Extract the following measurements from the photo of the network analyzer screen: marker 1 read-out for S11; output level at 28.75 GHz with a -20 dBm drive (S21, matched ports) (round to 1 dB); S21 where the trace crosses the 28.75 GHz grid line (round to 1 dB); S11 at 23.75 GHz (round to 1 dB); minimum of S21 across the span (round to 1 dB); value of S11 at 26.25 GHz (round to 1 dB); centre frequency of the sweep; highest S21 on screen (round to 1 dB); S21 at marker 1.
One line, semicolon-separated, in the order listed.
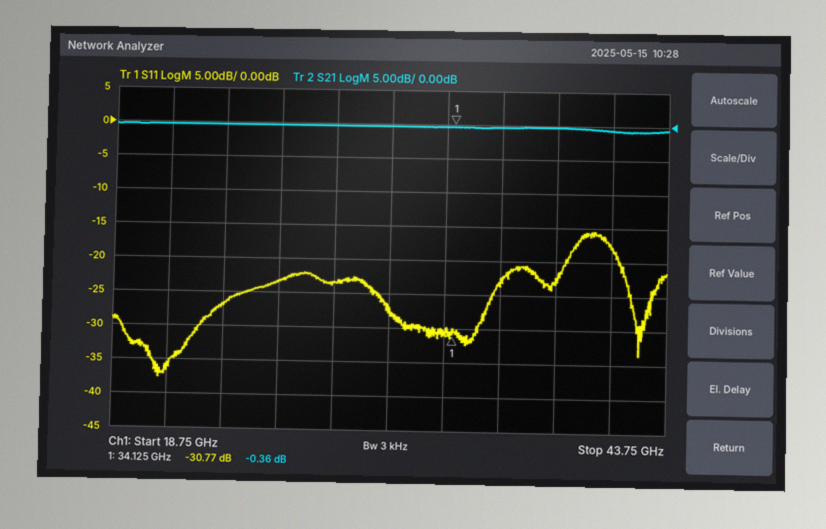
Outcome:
-30.77 dB; -20 dBm; 0 dB; -27 dB; -1 dB; -23 dB; 31.25 GHz; 0 dB; -0.36 dB
